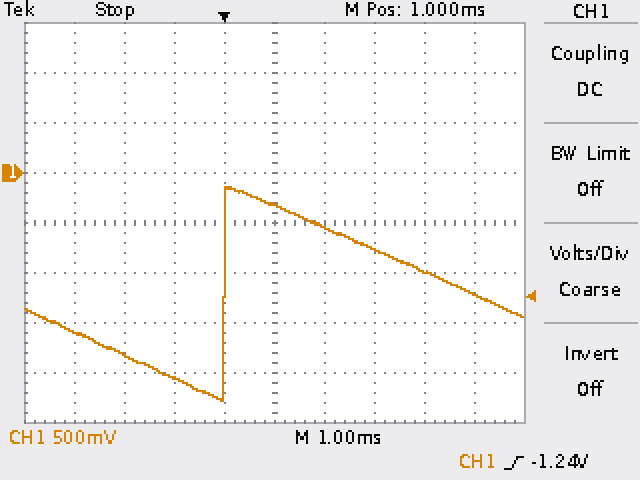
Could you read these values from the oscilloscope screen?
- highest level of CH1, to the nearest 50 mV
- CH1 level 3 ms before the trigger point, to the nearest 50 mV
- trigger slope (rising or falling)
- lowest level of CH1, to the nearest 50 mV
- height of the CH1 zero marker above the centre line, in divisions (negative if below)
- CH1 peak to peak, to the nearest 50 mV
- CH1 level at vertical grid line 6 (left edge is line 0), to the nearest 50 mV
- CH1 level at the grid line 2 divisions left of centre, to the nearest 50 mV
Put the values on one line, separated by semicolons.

-150 mV; -1.60 V; rising; -2.30 V; +1.0 div; 2.15 V; -550 mV; -2.05 V
